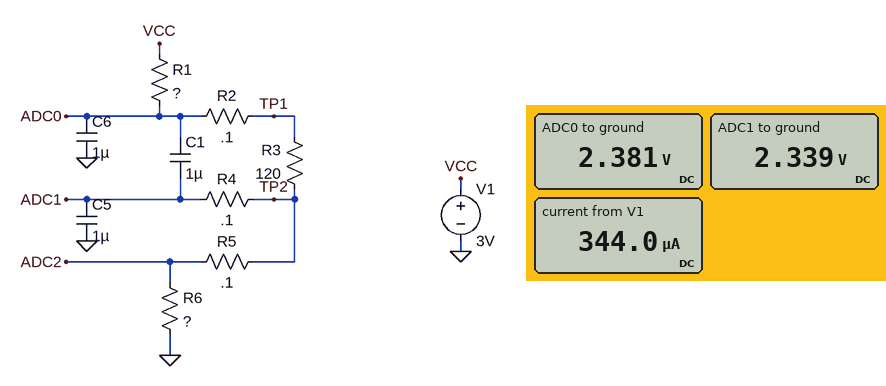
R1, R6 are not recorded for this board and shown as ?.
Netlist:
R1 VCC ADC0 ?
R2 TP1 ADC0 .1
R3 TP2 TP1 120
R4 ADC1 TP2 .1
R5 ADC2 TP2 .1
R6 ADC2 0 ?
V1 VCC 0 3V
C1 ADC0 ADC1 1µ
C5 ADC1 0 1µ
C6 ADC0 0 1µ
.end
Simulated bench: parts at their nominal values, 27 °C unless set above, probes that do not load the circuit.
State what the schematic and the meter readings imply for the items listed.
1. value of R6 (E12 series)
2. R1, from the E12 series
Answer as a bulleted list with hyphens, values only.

- 6.8 kΩ
- 1.8 kΩ
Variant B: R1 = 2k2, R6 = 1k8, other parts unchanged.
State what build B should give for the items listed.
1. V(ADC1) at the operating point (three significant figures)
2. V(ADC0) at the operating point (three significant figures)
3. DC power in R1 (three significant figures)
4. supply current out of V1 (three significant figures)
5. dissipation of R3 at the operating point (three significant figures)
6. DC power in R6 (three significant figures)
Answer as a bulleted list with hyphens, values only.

- 1.31 V
- 1.40 V
- 1.17 mW
- 728 µA
- 63.6 µW
- 954 µW
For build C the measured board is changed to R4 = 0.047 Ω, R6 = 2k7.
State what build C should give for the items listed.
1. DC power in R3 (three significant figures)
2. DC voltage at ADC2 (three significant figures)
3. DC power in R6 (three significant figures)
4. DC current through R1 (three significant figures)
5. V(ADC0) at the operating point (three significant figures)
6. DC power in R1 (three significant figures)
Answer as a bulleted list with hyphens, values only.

- 50.6 µW
- 1.75 V
- 1.14 mW
- 649 µA
- 1.83 V
- 759 µW
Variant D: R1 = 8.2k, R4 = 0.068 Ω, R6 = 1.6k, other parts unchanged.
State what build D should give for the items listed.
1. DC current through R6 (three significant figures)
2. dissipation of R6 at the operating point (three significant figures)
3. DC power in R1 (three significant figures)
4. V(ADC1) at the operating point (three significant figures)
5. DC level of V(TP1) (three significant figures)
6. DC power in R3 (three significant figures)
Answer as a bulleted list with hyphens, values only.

- 302 µA
- 146 µW
- 750 µW
- 484 mV
- 520 mV
- 11.0 µW
